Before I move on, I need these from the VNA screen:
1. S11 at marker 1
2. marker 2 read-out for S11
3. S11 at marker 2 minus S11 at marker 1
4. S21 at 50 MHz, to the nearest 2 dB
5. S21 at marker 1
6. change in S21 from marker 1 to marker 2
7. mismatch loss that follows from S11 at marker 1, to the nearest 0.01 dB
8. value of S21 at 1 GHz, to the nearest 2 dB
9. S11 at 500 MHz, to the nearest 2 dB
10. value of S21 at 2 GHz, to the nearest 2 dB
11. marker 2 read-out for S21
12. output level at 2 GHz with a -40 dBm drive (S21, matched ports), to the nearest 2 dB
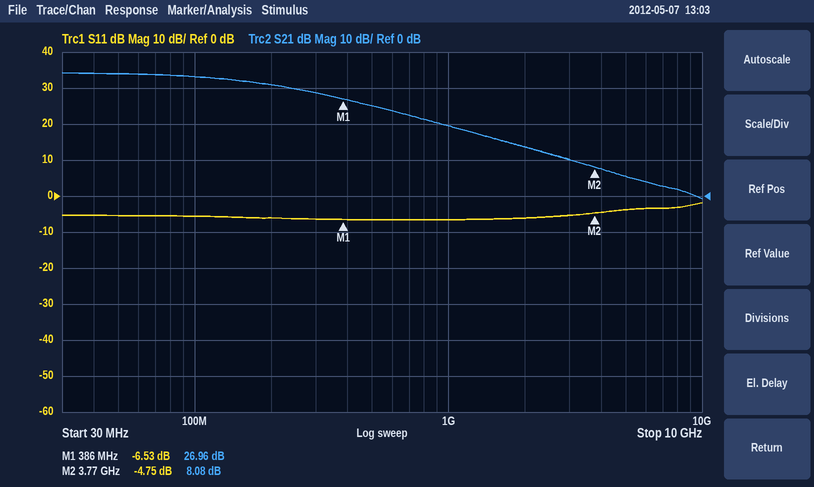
-6.53 dB
-4.75 dB
1.78 dB
34 dB
26.96 dB
-18.88 dB
1.09 dB
20 dB
-6 dB
14 dB
8.08 dB
-26 dBm
